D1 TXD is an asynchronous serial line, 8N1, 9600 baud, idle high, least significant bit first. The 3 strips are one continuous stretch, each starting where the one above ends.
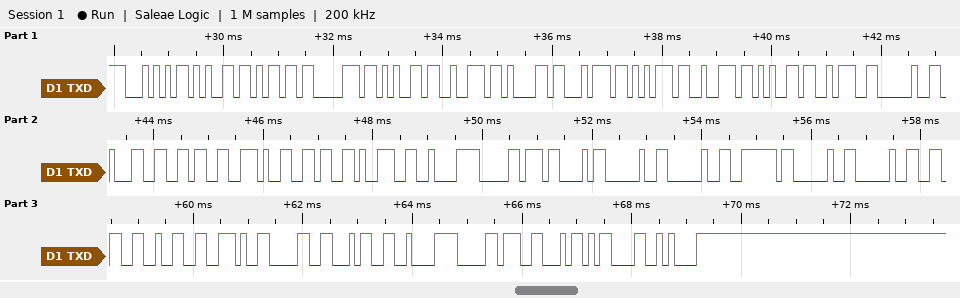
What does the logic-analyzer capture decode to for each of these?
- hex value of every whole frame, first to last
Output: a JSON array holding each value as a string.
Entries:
["54 65 6D 70 65 72 61 74 75 72 65 3A 20 31 36 2E 36 39 C2 B0 43 20 20 7E 20 20 36 32 2E 30 34 C2 B0 46 0D 0A"]
